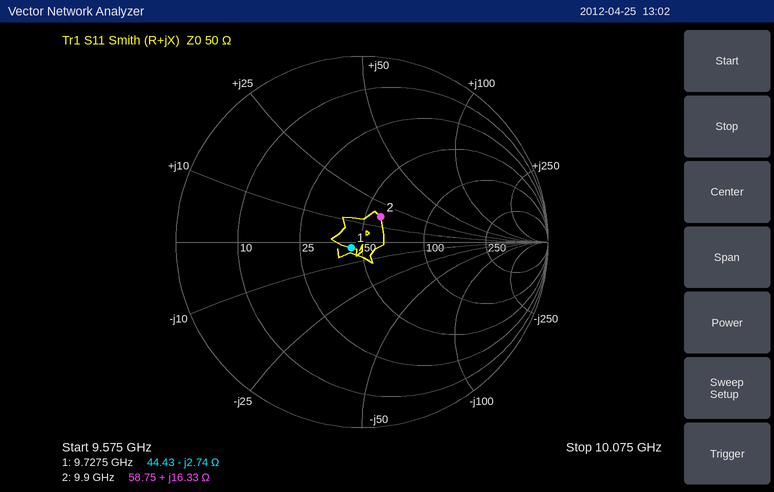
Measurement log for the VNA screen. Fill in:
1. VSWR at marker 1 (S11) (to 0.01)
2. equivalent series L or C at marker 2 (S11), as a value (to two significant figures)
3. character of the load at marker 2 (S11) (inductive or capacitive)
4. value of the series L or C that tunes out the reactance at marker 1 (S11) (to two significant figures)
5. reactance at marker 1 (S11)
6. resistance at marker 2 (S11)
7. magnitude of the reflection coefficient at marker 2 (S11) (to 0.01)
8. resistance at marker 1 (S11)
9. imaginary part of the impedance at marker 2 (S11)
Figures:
1.14
260 pH
inductive
45 pH
-2.74 Ω
58.75 Ω
0.17
44.43 Ω
+16.33 Ω
